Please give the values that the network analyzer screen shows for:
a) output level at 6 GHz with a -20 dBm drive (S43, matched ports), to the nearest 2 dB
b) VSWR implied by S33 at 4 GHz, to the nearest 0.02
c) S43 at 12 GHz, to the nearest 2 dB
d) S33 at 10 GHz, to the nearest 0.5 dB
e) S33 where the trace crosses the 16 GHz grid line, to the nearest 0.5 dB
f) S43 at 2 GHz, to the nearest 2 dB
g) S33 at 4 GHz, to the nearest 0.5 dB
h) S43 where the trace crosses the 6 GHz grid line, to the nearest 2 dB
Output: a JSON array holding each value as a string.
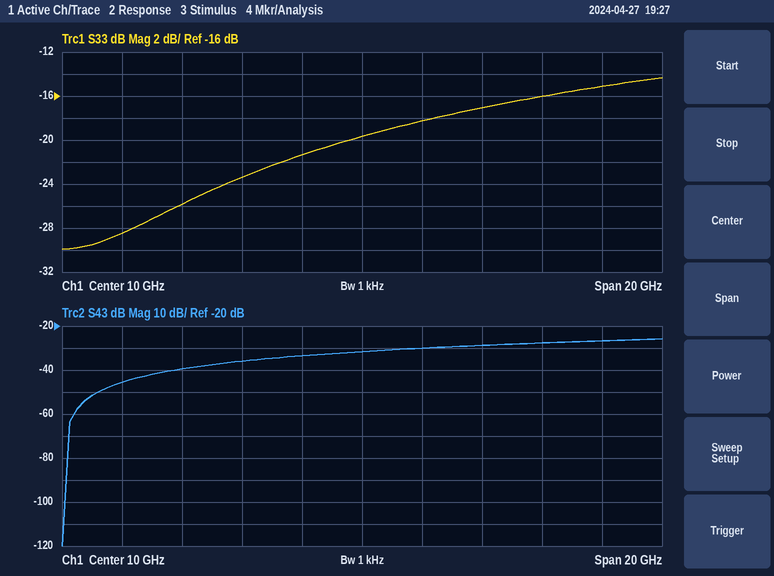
["-56 dBm", "1.10", "-30 dB", "-19.5 dB", "-16.0 dB", "-46 dB", "-26.0 dB", "-36 dB"]
